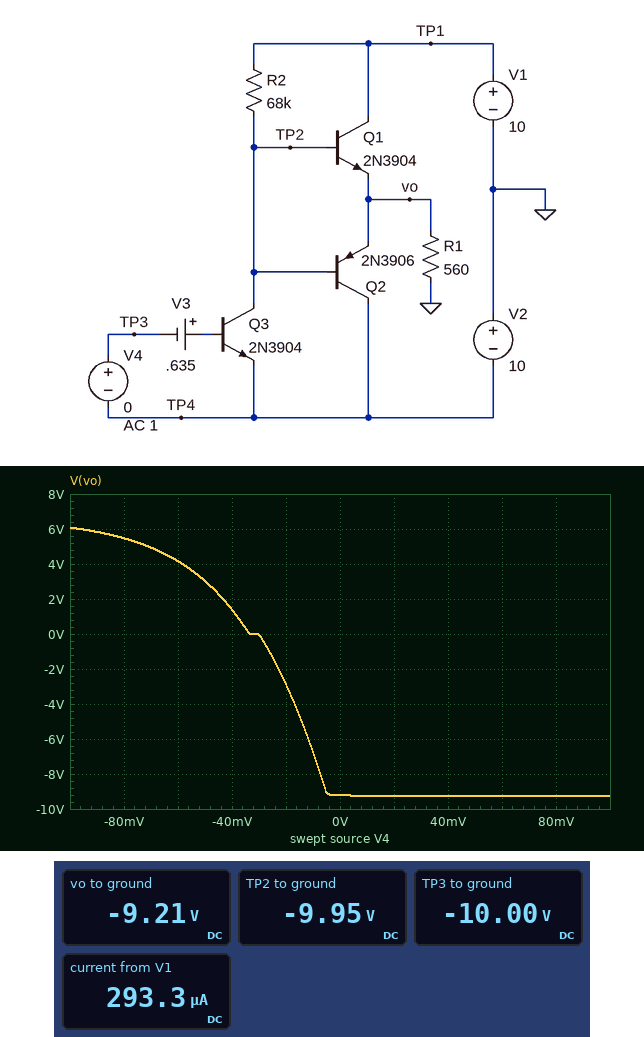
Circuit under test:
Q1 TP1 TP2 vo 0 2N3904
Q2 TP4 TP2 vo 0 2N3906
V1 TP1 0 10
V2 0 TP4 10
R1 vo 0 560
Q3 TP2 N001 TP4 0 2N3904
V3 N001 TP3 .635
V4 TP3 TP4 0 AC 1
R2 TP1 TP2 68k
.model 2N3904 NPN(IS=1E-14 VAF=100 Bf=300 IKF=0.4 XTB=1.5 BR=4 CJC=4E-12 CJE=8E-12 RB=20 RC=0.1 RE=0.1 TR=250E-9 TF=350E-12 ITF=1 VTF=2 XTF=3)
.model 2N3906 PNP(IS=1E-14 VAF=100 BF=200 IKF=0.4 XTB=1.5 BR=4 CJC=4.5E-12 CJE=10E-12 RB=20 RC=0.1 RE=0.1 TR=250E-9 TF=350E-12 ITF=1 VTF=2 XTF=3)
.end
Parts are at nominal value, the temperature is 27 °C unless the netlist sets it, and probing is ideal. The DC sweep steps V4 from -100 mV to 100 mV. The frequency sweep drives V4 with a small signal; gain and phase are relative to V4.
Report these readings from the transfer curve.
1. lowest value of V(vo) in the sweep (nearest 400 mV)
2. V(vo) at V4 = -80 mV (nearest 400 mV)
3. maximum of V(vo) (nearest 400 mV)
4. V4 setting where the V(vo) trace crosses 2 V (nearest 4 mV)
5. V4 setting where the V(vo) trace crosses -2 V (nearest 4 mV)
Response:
-9.2 V
5.6 V
6.0 V
-44 mV
-24 mV
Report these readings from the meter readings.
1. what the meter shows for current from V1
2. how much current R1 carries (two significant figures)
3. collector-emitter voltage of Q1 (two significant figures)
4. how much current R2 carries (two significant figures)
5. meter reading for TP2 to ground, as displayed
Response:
293.3 µA
16 mA
19 V
290 µA
-9.95 V
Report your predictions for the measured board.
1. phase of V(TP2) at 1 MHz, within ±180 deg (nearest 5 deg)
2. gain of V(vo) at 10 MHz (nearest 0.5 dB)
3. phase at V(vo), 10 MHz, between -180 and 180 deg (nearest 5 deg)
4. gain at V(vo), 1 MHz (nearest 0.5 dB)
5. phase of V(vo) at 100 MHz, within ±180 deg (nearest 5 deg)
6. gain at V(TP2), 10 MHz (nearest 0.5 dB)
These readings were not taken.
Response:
110 deg
-2.0 dB
25 deg
8.5 dB
-15 deg
-2.0 dB
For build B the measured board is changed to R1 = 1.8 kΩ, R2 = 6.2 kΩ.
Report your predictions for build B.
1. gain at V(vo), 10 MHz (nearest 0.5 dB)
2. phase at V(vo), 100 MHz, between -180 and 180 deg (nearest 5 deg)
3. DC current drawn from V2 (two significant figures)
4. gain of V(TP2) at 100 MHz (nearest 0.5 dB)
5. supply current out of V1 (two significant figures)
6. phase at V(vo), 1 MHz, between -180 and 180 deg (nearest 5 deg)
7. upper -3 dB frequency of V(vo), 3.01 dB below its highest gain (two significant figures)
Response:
33.5 dB
75 deg
530 µA
14.0 dB
3.8 mA
165 deg
4.3 MHz
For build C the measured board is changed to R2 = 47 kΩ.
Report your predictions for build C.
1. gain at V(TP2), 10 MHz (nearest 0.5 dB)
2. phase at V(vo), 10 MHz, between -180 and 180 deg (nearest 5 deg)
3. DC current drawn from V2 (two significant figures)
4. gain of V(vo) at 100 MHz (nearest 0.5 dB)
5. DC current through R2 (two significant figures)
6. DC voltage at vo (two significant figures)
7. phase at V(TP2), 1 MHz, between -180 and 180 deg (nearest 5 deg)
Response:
29.5 dB
90 deg
14 mA
9.5 dB
390 µA
-7.7 V
120 deg
